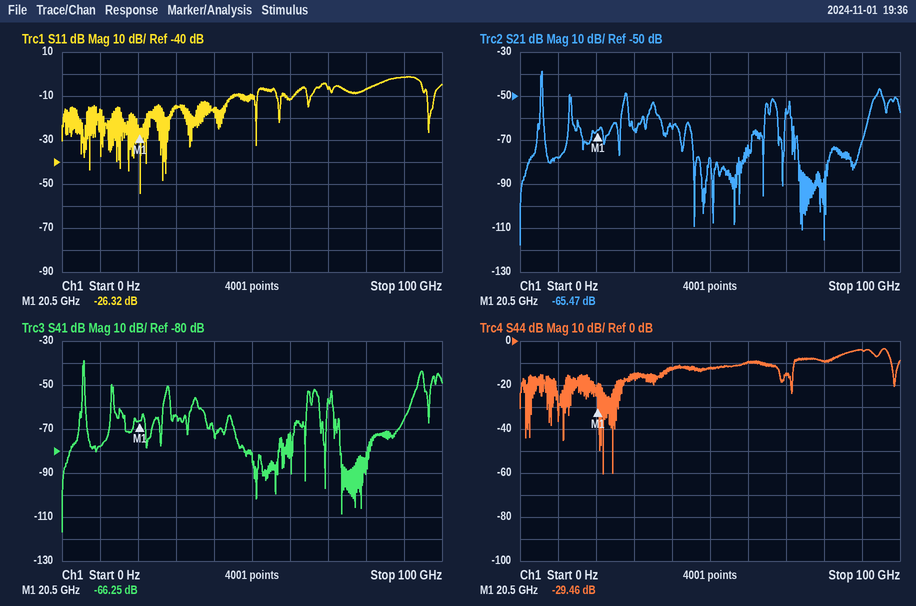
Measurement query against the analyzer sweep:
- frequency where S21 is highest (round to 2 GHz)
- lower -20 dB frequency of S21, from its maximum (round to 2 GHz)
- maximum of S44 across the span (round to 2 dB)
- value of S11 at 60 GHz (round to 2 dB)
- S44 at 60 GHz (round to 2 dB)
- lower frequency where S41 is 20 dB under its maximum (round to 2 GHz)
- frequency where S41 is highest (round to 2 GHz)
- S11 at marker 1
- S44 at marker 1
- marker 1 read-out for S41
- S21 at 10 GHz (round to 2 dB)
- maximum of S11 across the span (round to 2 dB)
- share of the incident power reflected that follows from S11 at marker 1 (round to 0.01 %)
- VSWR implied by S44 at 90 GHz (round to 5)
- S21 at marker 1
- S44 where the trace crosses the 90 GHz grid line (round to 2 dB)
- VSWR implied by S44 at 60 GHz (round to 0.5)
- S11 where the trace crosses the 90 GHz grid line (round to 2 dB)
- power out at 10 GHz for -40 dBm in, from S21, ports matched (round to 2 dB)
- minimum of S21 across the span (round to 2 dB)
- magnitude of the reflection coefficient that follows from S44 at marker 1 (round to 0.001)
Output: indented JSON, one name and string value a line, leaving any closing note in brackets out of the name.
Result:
{
  "frequency where S21 is highest": "6 GHz",
  "lower -20 dB frequency of S21, from its maximum": "6 GHz",
  "maximum of S44 across the span": "-4 dB",
  "value of S11 at 60 GHz": "-12 dB",
  "S44 at 60 GHz": "-10 dB",
  "lower frequency where S41 is 20 dB under its maximum": "6 GHz",
  "frequency where S41 is highest": "6 GHz",
  "S11 at marker 1": "-26.32 dB",
  "S44 at marker 1": "-29.46 dB",
  "marker 1 read-out for S41": "-66.25 dB",
  "S21 at 10 GHz": "-78 dB",
  "maximum of S11 across the span": "-2 dB",
  "share of the incident power reflected that follows from S11 at marker 1": "0.23 %",
  "VSWR implied by S44 at 90 GHz": "5",
  "S21 at marker 1": "-65.47 dB",
  "S44 where the trace crosses the 90 GHz grid line": "-4 dB",
  "VSWR implied by S44 at 60 GHz": "2.0",
  "S11 where the trace crosses the 90 GHz grid line": "-2 dB",
  "power out at 10 GHz for -40 dBm in, from S21, ports matched": "-118 dBm",
  "minimum of S21 across the span": "-118 dB",
  "magnitude of the reflection coefficient that follows from S44 at marker 1": "0.034"
}
